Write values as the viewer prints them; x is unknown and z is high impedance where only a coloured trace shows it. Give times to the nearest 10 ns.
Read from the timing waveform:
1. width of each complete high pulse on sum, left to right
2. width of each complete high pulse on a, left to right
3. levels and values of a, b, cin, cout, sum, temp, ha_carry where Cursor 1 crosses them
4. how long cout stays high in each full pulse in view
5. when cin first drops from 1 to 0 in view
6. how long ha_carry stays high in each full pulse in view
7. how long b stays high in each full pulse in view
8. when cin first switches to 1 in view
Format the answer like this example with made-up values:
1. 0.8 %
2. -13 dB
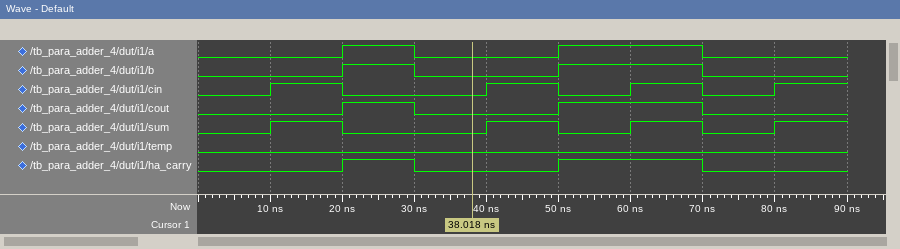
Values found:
1. 10 ns, 10 ns, 10 ns
2. 10 ns, 20 ns
3. a=0, b=0, cin=0, cout=0, sum=0, temp=0, ha_carry=0
4. 10 ns, 20 ns
5. 20 ns
6. 10 ns, 20 ns
7. 10 ns, 20 ns
8. 10 ns
